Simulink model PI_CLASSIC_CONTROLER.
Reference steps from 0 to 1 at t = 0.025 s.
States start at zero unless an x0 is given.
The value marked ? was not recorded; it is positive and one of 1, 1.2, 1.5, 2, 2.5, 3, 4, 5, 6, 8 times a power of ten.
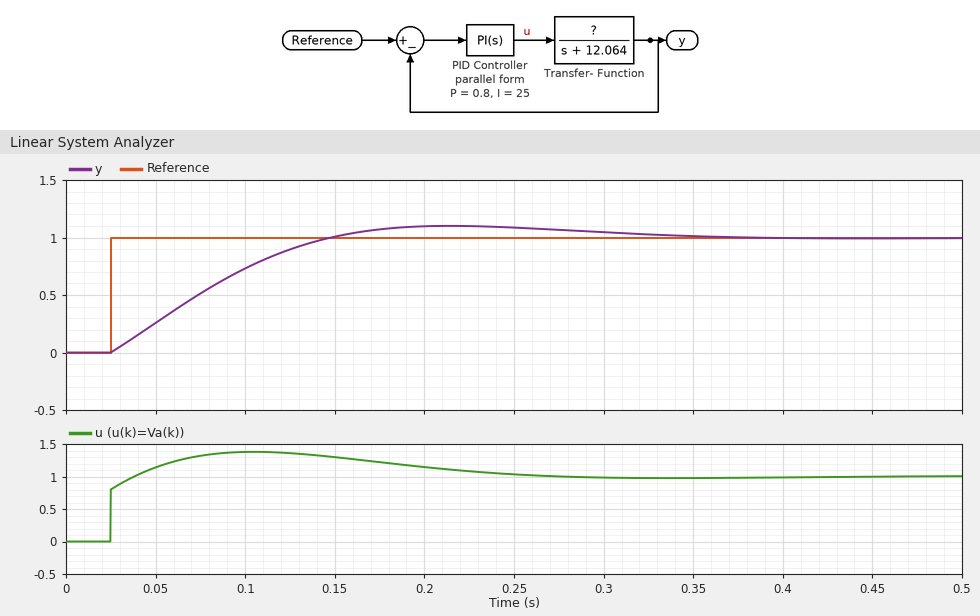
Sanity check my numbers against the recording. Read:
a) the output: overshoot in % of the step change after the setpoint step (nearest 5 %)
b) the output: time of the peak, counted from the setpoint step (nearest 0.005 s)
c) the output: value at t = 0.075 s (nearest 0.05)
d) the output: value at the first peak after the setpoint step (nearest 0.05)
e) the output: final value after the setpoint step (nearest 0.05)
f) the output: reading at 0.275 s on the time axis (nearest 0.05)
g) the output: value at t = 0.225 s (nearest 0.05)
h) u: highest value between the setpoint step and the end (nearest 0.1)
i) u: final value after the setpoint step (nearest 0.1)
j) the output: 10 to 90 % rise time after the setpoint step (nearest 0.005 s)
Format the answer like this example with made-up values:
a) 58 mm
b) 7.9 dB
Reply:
a) 10 %
b) 0.190 s
c) 0.50
d) 1.10
e) 1.00
f) 1.05
g) 1.10
h) 1.4
i) 1.0
j) 0.090 s
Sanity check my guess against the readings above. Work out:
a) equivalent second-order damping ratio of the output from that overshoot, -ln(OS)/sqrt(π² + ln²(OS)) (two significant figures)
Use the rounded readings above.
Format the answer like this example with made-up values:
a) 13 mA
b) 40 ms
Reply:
a) 0.59
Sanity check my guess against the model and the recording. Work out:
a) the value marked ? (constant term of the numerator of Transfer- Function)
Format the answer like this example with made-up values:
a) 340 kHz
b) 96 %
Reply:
a) 12
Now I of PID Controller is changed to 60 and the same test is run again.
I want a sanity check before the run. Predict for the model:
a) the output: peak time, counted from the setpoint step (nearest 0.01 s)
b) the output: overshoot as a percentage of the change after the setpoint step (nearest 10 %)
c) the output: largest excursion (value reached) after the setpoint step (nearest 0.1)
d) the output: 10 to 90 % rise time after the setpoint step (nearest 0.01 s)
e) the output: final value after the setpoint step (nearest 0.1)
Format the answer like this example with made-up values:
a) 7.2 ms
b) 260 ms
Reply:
a) 0.11 s
b) 30 %
c) 1.3
d) 0.05 s
e) 1.0
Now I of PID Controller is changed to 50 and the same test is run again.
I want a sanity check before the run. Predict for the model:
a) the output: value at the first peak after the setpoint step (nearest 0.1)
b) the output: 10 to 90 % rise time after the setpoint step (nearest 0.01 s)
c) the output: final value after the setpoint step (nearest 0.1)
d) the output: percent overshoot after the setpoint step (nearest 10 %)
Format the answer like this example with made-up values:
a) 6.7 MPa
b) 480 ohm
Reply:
a) 1.2
b) 0.06 s
c) 1.0
d) 20 %
